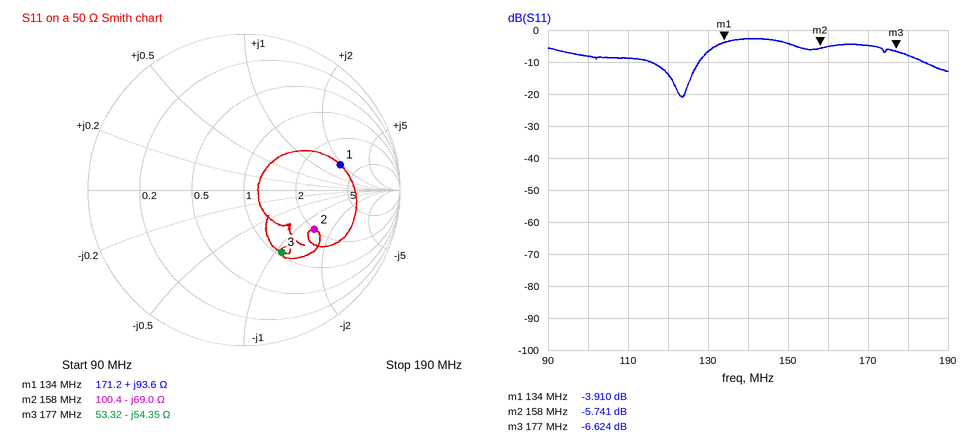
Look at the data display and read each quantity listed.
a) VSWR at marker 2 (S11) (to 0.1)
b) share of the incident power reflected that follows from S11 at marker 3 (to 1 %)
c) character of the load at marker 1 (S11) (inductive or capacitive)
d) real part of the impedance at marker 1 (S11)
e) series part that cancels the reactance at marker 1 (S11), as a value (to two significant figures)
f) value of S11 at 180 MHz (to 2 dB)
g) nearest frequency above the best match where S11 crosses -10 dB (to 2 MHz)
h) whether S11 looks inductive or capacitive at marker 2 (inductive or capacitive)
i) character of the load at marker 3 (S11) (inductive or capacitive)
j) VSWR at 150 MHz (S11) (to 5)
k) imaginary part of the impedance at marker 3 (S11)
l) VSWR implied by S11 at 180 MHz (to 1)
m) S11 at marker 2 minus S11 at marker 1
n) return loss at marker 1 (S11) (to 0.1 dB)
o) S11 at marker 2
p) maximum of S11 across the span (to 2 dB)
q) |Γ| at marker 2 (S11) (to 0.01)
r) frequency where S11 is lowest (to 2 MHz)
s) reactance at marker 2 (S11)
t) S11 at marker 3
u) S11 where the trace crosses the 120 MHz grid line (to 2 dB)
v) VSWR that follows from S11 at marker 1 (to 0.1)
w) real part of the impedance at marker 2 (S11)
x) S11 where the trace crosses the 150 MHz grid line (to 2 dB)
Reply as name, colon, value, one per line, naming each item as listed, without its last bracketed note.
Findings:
VSWR at marker 2 (S11): 3.1
share of the incident power reflected that follows from S11 at marker 3: 22 %
character of the load at marker 1 (S11): inductive
real part of the impedance at marker 1: 171.2 Ω
series part that cancels the reactance at marker 1 (S11), as a value: 13 pF
value of S11 at 180 MHz: -8 dB
nearest frequency above the best match where S11 crosses -10 dB: 128 MHz
whether S11 looks inductive or capacitive at marker 2: capacitive
character of the load at marker 3 (S11): capacitive
VSWR at 150 MHz (S11): 5
imaginary part of the impedance at marker 3: -54.35 Ω
VSWR implied by S11 at 180 MHz: 2
S11 at marker 2 minus S11 at marker 1: -1.831 dB
return loss at marker 1 (S11): 3.9 dB
S11 at marker 2: -5.741 dB
maximum of S11 across the span: -2 dB
|Γ| at marker 2 (S11): 0.52
frequency where S11 is lowest: 124 MHz
reactance at marker 2: -69.0 Ω
S11 at marker 3: -6.624 dB
S11 where the trace crosses the 120 MHz grid line: -14 dB
VSWR that follows from S11 at marker 1: 4.5
real part of the impedance at marker 2: 100.4 Ω
S11 where the trace crosses the 150 MHz grid line: -4 dB
